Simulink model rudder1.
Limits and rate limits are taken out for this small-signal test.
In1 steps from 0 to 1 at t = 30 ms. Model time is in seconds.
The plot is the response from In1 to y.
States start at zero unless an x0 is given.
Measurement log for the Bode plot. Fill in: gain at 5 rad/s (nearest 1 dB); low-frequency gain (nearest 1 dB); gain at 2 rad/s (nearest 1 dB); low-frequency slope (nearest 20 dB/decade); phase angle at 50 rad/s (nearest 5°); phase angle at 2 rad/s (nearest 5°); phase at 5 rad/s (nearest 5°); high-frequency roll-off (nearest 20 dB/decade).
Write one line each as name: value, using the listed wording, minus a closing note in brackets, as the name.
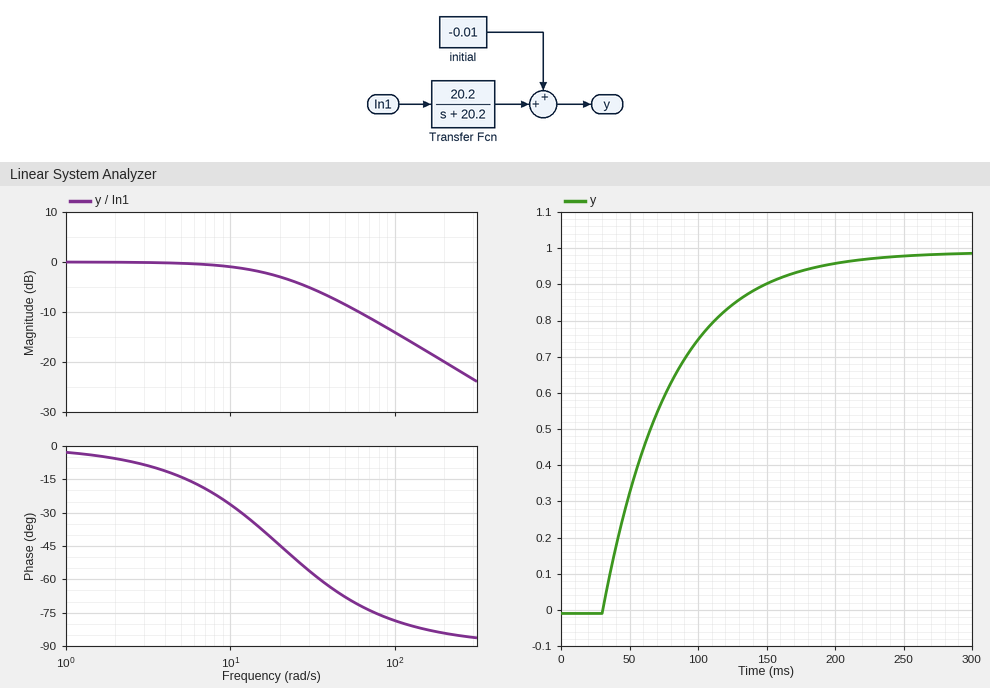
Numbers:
gain at 5 rad/s: 0 dB
low-frequency gain: 0 dB
gain at 2 rad/s: 0 dB
low-frequency slope: 0 dB/decade
phase angle at 50 rad/s: -70°
phase angle at 2 rad/s: -5°
phase at 5 rad/s: -15°
high-frequency roll-off: -20 dB/decade
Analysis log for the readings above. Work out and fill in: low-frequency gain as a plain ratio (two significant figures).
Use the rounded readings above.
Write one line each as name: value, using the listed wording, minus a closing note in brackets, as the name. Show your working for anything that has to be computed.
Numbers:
low-frequency gain as a plain ratio: 10^(0 / 20) = 1.0
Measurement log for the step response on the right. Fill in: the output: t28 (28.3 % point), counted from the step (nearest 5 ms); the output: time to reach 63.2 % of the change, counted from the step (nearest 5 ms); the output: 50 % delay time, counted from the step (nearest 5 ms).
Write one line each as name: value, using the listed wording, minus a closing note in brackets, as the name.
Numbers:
the output: t28 (28.3 % point), counted from the step: 15 ms
the output: time to reach 63.2 % of the change, counted from the step: 50 ms
the output: 50 % delay time, counted from the step: 35 ms
